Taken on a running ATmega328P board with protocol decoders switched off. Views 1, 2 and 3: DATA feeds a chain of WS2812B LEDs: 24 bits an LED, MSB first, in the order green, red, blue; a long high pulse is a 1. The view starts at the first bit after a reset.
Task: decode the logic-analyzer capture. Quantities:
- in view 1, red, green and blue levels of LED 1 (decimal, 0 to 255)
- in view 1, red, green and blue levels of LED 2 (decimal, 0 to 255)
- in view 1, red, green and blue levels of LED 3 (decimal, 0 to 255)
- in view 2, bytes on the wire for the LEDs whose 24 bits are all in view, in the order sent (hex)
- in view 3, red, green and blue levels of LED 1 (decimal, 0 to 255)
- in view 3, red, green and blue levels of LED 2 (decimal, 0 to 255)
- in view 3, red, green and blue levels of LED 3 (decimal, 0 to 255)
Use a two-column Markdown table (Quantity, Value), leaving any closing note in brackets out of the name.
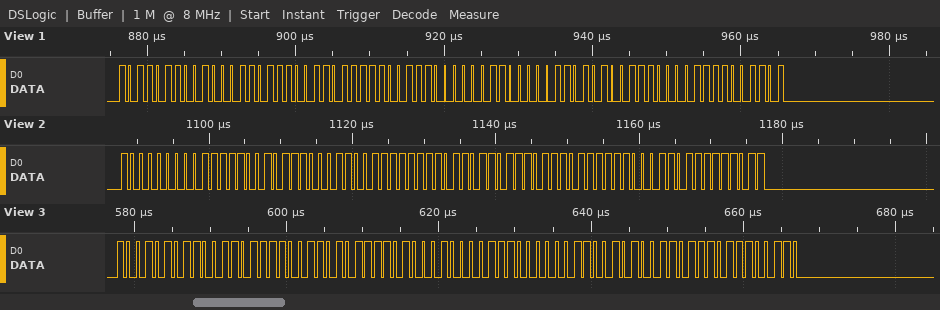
| Quantity | Value |
|---|---|
| in view 1, red, green and blue levels of LED 1 | 70, 182, 230 |
| in view 1, red, green and blue levels of LED 2 | 192, 249, 193 |
| in view 1, red, green and blue levels of LED 3 | 195, 169, 205 |
| in view 2, bytes on the wire for the LEDs whose 24 bits are all in view, in the order sent | 80 7C B8 CF F6 DD DF 8D FB |
| in view 3, red, green and blue levels of LED 1 | 155, 149, 205 |
| in view 3, red, green and blue levels of LED 2 | 33, 122, 192 |
| in view 3, red, green and blue levels of LED 3 | 110, 202, 230 |
